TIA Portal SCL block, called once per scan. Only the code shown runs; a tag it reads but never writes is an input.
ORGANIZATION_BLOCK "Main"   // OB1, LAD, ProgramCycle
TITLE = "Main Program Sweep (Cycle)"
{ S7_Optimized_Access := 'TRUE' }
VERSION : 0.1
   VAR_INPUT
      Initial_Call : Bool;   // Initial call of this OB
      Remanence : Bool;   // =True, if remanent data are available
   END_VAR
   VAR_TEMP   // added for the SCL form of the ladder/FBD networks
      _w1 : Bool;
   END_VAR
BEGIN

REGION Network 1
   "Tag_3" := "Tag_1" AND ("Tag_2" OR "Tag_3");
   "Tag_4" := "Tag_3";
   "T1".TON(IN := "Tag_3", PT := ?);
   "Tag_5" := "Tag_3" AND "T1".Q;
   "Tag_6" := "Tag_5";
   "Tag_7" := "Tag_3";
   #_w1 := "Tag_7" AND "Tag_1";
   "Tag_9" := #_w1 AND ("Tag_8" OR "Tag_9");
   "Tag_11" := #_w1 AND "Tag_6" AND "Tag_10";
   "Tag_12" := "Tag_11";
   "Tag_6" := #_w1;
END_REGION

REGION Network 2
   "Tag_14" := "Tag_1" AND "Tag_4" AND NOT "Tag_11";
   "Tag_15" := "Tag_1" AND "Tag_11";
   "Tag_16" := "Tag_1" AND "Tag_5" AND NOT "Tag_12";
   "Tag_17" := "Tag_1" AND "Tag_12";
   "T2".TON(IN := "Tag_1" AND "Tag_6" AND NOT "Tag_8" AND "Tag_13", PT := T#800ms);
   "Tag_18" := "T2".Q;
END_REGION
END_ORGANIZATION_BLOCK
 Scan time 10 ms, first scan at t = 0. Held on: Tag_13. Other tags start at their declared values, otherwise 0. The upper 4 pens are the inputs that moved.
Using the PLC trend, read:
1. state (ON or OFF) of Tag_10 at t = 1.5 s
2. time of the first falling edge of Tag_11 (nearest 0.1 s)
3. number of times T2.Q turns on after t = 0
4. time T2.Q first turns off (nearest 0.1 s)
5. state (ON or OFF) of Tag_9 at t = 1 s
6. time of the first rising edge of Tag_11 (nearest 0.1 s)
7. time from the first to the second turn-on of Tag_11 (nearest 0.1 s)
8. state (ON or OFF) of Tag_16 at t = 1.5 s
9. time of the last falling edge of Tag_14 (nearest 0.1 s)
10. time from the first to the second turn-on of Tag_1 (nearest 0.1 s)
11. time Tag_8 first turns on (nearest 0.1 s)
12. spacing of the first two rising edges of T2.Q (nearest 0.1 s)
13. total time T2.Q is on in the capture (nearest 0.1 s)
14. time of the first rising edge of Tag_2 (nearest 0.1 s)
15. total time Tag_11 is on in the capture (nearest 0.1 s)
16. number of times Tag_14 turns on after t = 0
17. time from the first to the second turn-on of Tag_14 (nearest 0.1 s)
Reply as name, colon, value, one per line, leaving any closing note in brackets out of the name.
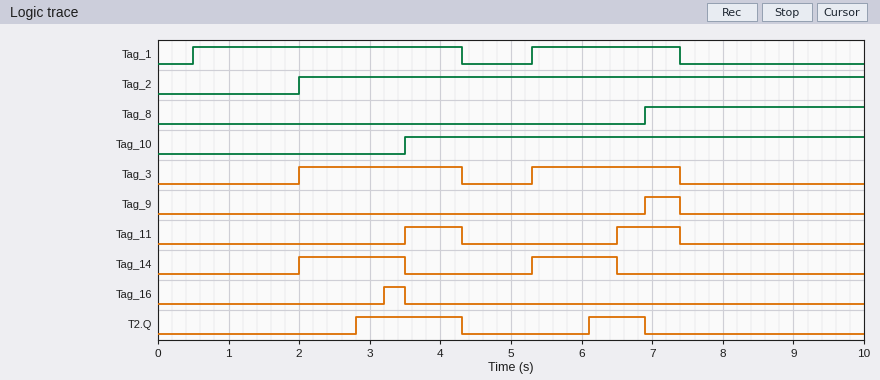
state (ON or OFF) of Tag_10 at t = 1.5 s: OFF
time of the first falling edge of Tag_11: 4.3 s
number of times T2.Q turns on after t = 0: 2
time T2.Q first turns off: 4.3 s
state (ON or OFF) of Tag_9 at t = 1 s: OFF
time of the first rising edge of Tag_11: 3.5 s
time from the first to the second turn-on of Tag_11: 3.0 s
state (ON or OFF) of Tag_16 at t = 1.5 s: OFF
time of the last falling edge of Tag_14: 6.5 s
time from the first to the second turn-on of Tag_1: 4.8 s
time Tag_8 first turns on: 6.9 s
spacing of the first two rising edges of T2.Q: 3.3 s
total time T2.Q is on in the capture: 2.3 s
time of the first rising edge of Tag_2: 2.0 s
total time Tag_11 is on in the capture: 1.7 s
number of times Tag_14 turns on after t = 0: 2
time from the first to the second turn-on of Tag_14: 3.3 s
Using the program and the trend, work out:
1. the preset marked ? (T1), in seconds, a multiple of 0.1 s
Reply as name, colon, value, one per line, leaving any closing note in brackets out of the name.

the preset marked ? (T1), in seconds, a multiple of 0.1 s: 1.2 s
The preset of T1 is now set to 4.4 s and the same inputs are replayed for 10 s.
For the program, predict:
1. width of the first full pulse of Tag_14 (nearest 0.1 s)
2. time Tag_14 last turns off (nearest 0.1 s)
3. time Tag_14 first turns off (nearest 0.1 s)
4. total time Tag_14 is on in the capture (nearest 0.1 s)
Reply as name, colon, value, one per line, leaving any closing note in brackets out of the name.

width of the first full pulse of Tag_14: 2.3 s
time Tag_14 last turns off: 7.4 s
time Tag_14 first turns off: 4.3 s
total time Tag_14 is on in the capture: 4.4 s
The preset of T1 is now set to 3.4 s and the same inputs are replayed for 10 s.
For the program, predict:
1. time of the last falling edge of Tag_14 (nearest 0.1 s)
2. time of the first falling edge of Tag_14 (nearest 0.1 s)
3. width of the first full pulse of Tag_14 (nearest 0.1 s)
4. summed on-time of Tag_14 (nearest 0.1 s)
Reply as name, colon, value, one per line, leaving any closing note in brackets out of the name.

time of the last falling edge of Tag_14: 7.4 s
time of the first falling edge of Tag_14: 4.3 s
width of the first full pulse of Tag_14: 2.3 s
summed on-time of Tag_14: 4.4 s
